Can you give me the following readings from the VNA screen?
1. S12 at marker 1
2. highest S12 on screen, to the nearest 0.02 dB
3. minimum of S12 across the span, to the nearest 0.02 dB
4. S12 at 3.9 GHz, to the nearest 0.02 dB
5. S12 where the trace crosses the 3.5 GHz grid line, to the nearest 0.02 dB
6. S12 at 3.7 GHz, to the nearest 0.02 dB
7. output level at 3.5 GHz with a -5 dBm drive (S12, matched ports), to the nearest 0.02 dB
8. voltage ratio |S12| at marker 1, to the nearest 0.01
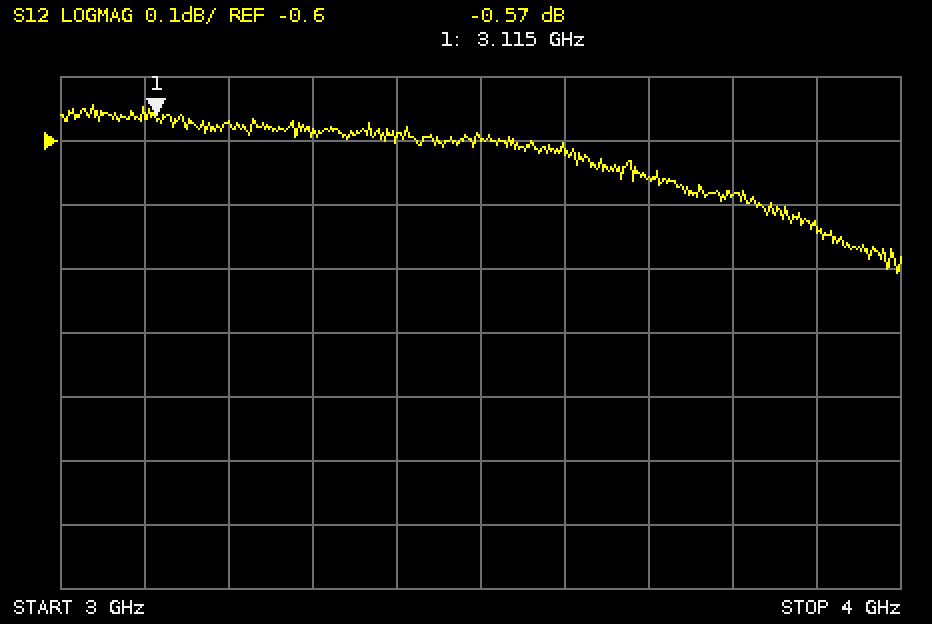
-0.57 dB
-0.54 dB
-0.80 dB
-0.74 dB
-0.60 dB
-0.66 dB
-5.60 dBm
0.94
